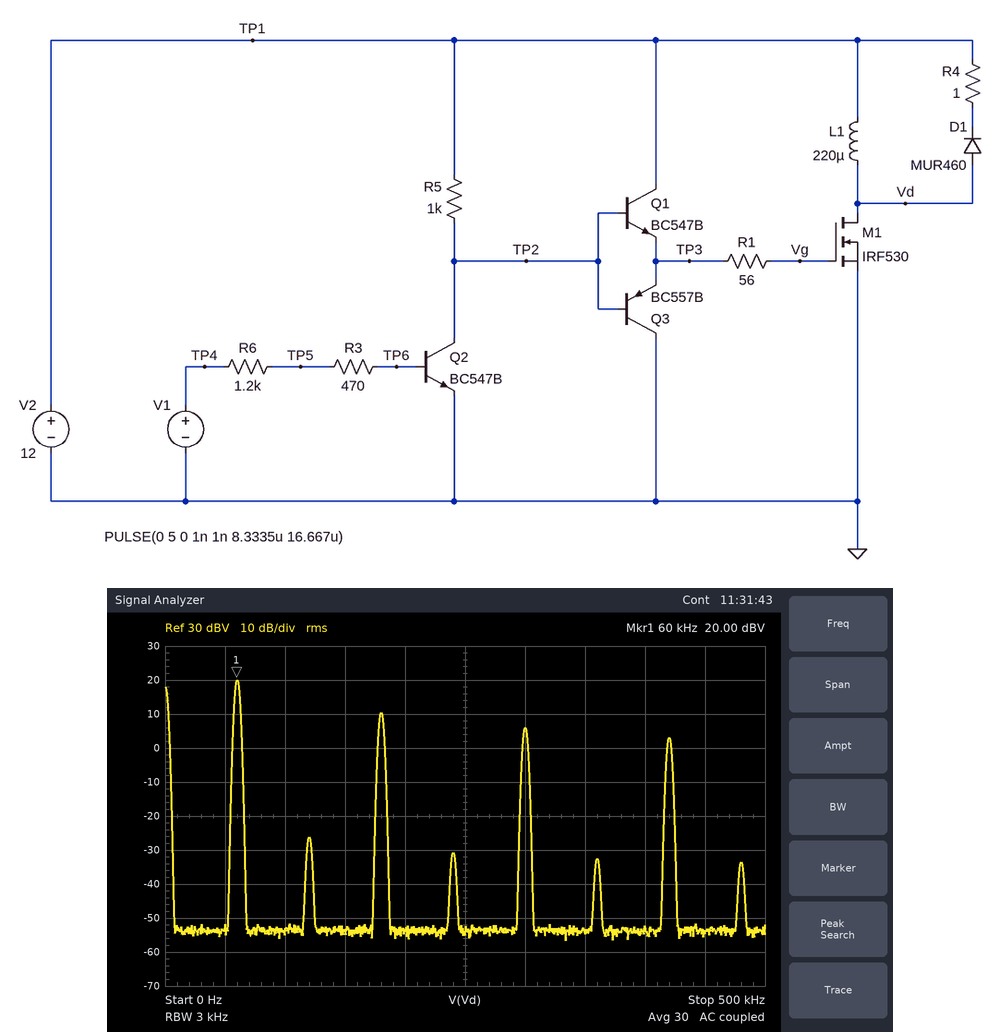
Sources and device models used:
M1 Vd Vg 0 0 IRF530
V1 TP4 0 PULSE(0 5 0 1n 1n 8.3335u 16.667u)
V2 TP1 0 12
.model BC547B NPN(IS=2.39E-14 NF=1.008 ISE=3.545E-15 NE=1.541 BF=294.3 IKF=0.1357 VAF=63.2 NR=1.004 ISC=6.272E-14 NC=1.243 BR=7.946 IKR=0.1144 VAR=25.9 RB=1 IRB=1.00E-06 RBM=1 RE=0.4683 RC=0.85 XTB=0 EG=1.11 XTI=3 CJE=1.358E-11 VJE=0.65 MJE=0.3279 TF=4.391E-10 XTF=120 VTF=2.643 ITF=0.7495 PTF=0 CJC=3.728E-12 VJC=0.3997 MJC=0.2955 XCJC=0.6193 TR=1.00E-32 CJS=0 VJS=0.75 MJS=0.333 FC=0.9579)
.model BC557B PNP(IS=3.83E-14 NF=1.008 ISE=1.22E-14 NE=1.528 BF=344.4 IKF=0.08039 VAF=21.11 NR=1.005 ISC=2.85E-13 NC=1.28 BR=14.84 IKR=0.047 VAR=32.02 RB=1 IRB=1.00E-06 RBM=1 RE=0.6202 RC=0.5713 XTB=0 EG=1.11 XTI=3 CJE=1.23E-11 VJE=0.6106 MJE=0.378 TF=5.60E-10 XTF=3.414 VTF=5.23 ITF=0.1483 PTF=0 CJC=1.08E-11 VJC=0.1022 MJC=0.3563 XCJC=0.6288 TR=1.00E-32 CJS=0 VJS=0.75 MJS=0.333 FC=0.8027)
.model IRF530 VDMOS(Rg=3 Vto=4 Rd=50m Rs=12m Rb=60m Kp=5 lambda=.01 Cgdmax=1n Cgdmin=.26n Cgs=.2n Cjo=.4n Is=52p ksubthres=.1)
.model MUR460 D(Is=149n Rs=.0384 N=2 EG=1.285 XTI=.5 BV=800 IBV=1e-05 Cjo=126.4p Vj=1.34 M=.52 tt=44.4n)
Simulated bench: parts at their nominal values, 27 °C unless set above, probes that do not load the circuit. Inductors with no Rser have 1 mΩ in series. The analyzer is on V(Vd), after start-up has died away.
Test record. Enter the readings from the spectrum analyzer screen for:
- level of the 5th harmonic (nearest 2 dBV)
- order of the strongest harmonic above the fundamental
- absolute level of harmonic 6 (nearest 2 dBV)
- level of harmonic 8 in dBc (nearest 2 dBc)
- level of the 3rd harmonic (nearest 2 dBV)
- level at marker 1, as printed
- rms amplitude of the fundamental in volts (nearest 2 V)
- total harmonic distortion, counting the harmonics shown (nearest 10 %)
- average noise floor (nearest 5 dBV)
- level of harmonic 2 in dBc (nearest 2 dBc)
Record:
6 dBV
3
-32 dBV
-54 dBc
10 dBV
20.00 dBV
10 V
40 %
-55 dBV
-46 dBc
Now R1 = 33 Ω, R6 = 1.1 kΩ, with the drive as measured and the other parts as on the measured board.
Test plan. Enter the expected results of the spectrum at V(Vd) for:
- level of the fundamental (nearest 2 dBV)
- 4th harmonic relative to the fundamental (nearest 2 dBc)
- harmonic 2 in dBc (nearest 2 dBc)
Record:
20 dBV
-42 dBc
-42 dBc
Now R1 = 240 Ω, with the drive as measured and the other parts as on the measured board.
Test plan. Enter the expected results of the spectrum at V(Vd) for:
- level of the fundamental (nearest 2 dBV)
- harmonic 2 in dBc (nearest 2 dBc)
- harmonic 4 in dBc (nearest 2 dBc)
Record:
20 dBV
-28 dBc
-28 dBc
